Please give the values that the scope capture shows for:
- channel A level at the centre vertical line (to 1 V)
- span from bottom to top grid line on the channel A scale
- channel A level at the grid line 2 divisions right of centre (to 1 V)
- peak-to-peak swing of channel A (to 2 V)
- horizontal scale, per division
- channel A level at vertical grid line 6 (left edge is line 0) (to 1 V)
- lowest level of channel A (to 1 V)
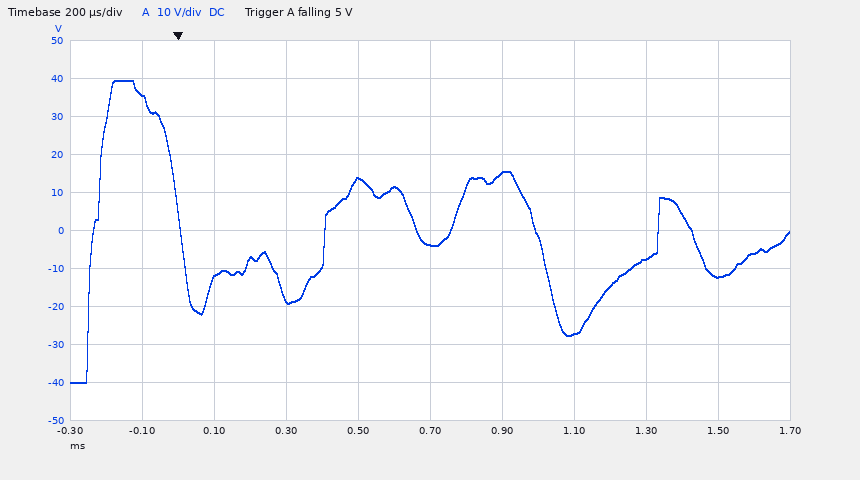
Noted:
-4 V
100 V
-27 V
80 V
200 µs
15 V
-40 V
